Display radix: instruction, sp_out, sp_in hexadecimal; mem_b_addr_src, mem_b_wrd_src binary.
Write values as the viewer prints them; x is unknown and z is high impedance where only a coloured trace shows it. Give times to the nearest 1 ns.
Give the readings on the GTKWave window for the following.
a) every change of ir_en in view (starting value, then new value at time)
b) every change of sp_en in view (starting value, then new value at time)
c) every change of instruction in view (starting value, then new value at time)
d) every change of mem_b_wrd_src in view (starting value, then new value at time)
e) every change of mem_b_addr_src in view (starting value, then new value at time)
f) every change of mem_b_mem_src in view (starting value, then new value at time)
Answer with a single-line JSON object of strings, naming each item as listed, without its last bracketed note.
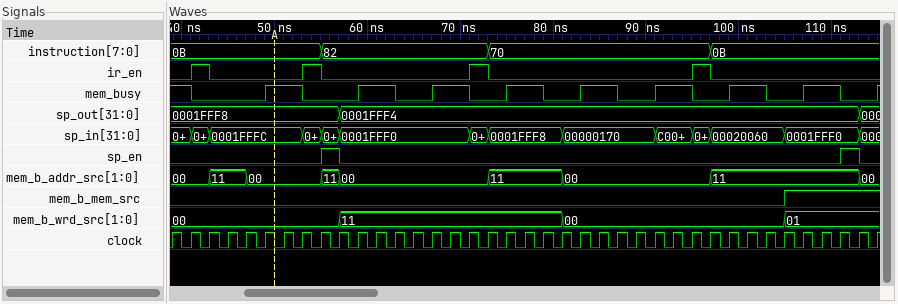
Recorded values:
{"every change of ir_en in view": "0, 1 at 41 ns, 0 at 43 ns, 1 at 53 ns, 0 at 55 ns, 1 at 71 ns, 0 at 73 ns, 1 at 95 ns, 0 at 97 ns", "every change of sp_en in view": "0, 1 at 55 ns, 0 at 57 ns, 1 at 111 ns, 0 at 113 ns", "every change of instruction in view": "0B, 82 at 55 ns, 70 at 73 ns, 0B at 97 ns", "every change of mem_b_wrd_src in view": "00, 11 at 57 ns, 00 at 81 ns, 01 at 105 ns", "every change of mem_b_addr_src in view": "00, 11 at 43 ns, 00 at 47 ns, 11 at 55 ns, 00 at 57 ns, 11 at 73 ns, 00 at 81 ns, 11 at 97 ns, 00 at 113 ns", "every change of mem_b_mem_src in view": "0, 1 at 105 ns"}
